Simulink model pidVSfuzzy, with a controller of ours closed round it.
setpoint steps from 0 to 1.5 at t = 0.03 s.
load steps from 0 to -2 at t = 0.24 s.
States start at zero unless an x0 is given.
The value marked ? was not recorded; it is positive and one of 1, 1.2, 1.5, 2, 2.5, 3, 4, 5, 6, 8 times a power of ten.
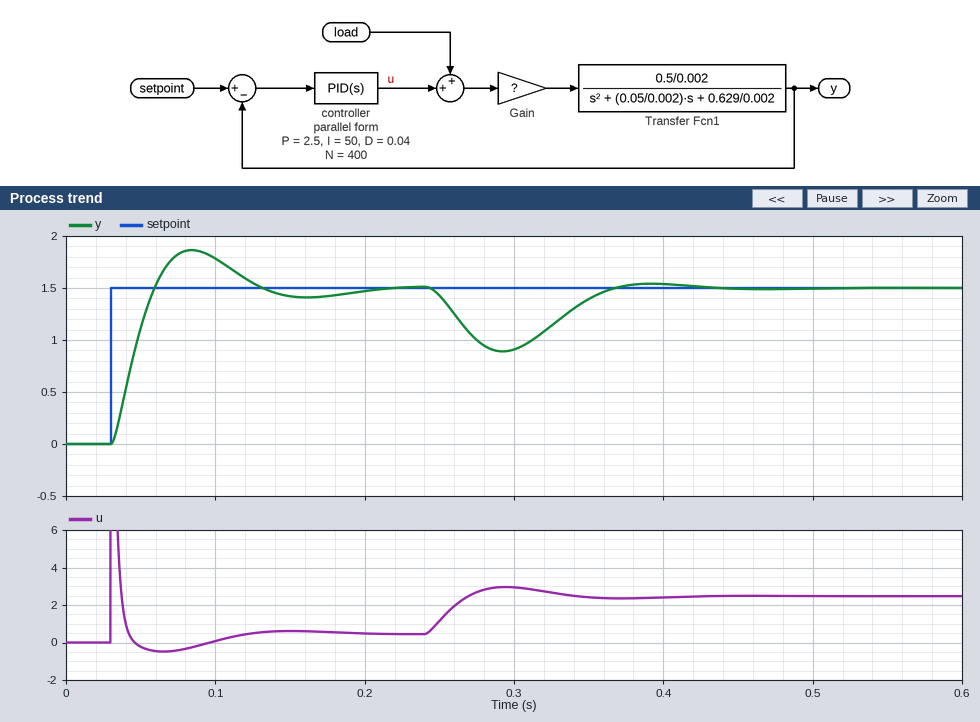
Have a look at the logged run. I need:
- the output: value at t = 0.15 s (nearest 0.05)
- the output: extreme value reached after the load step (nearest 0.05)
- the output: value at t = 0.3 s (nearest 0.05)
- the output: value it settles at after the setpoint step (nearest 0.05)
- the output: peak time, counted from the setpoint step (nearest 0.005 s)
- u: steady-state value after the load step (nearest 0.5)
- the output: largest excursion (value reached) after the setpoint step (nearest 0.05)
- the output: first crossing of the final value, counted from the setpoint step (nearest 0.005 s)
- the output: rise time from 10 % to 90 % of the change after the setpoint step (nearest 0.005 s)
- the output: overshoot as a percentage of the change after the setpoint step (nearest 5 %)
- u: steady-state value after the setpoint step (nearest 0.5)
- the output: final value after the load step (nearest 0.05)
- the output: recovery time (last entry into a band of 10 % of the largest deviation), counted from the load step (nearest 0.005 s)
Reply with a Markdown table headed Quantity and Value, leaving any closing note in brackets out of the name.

| Quantity | Value |
|---|---|
| the output: value at t = 0.15 s | 1.40 |
| the output: extreme value reached after the load step | 0.90 |
| the output: value at t = 0.3 s | 0.90 |
| the output: value it settles at after the setpoint step | 1.50 |
| the output: peak time, counted from the setpoint step | 0.055 s |
| u: steady-state value after the load step | 2.5 |
| the output: largest excursion (value reached) after the setpoint step | 1.85 |
| the output: first crossing of the final value, counted from the setpoint step | 0.030 s |
| the output: rise time from 10 % to 90 % of the change after the setpoint step | 0.020 s |
| the output: overshoot as a percentage of the change after the setpoint step | 25 % |
| u: steady-state value after the setpoint step | 0.5 |
| the output: final value after the load step | 1.50 |
| the output: recovery time (last entry into a band of 10 % of the largest deviation), counted from the load step | 0.115 s |
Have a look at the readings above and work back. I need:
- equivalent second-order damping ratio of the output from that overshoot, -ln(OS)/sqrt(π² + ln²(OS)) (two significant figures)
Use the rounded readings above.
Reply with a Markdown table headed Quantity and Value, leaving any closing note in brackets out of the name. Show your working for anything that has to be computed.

| Quantity | Value |
|---|---|
| equivalent second-order damping ratio of the output from that overshoot, -ln(OS)/sqrt(π² + ln²(OS)) | ln(0.25) = -1.386; 1.386 / sqrt(9.870 + 1.922) = 0.40 |
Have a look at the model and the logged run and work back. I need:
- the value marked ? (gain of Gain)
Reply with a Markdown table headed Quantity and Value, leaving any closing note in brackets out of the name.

| Quantity | Value |
|---|---|
| the value marked ? | 4 |
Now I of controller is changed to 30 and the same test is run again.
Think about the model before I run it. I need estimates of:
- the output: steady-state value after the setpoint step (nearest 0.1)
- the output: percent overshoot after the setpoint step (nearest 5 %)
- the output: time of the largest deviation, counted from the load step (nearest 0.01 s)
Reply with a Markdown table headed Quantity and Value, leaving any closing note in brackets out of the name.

| Quantity | Value |
|---|---|
| the output: steady-state value after the setpoint step | 1.5 |
| the output: percent overshoot after the setpoint step | 15 % |
| the output: time of the largest deviation, counted from the load step | 0.06 s |
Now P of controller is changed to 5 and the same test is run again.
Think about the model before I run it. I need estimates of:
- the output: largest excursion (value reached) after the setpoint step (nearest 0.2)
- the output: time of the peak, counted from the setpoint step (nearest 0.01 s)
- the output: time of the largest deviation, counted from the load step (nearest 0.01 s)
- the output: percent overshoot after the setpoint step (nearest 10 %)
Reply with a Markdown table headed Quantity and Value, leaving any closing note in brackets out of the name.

| Quantity | Value |
|---|---|
| the output: largest excursion (value reached) after the setpoint step | 2.0 |
| the output: time of the peak, counted from the setpoint step | 0.04 s |
| the output: time of the largest deviation, counted from the load step | 0.04 s |
| the output: percent overshoot after the setpoint step | 30 % |
